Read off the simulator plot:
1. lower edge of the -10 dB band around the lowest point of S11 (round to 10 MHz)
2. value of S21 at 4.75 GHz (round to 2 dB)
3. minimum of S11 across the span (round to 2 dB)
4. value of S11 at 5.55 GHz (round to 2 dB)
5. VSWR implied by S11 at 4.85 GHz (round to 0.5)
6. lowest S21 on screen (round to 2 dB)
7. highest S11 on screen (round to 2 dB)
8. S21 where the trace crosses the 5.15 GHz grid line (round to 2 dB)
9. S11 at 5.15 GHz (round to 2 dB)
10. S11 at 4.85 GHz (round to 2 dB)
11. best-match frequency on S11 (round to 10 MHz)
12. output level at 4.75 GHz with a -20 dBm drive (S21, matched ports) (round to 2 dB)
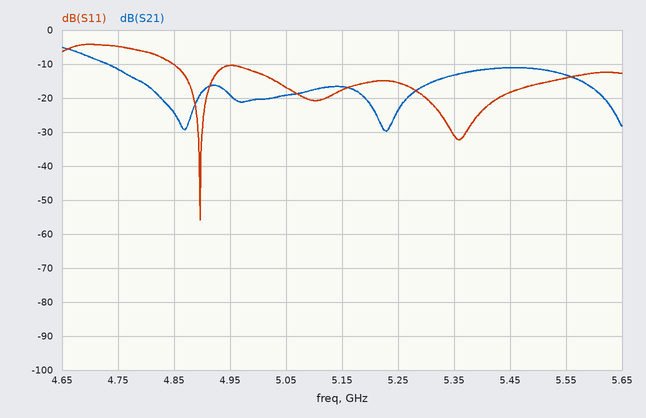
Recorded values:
4.85 GHz
-12 dB
-56 dB
-14 dB
2.0
-30 dB
-4 dB
-16 dB
-18 dB
-10 dB
4.90 GHz
-32 dBm
